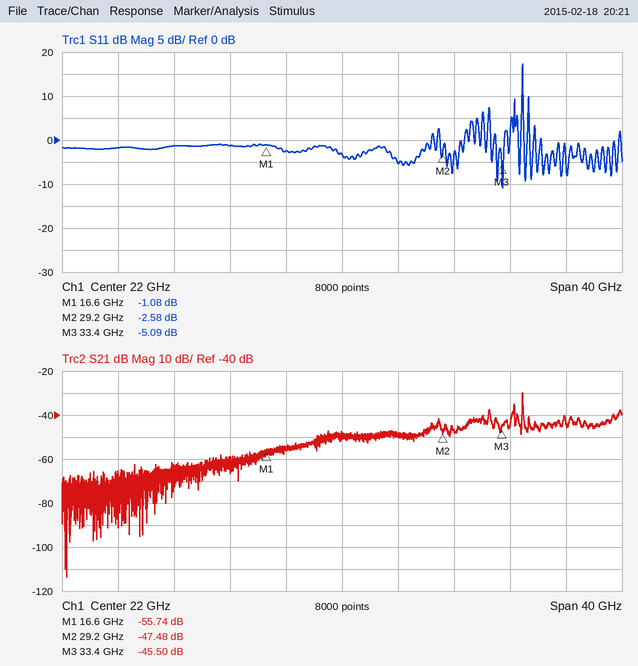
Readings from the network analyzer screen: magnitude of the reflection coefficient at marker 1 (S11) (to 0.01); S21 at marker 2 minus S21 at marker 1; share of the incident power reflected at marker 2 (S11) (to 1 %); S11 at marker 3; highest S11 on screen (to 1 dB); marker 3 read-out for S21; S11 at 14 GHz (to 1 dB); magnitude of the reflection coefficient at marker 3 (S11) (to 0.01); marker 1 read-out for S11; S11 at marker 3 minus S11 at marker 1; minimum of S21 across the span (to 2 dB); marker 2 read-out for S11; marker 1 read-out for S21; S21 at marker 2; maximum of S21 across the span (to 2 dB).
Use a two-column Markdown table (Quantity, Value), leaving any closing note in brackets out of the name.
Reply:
| Quantity | Value |
|---|---|
| magnitude of the reflection coefficient at marker 1 (S11) | 0.88 |
| S21 at marker 2 minus S21 at marker 1 | 8.26 dB |
| share of the incident power reflected at marker 2 (S11) | 55 % |
| S11 at marker 3 | -5.09 dB |
| highest S11 on screen | 17 dB |
| marker 3 read-out for S21 | -45.50 dB |
| S11 at 14 GHz | -1 dB |
| magnitude of the reflection coefficient at marker 3 (S11) | 0.56 |
| marker 1 read-out for S11 | -1.08 dB |
| S11 at marker 3 minus S11 at marker 1 | -4.01 dB |
| minimum of S21 across the span | -114 dB |
| marker 2 read-out for S11 | -2.58 dB |
| marker 1 read-out for S21 | -55.74 dB |
| S21 at marker 2 | -47.48 dB |
| maximum of S21 across the span | -30 dB |
